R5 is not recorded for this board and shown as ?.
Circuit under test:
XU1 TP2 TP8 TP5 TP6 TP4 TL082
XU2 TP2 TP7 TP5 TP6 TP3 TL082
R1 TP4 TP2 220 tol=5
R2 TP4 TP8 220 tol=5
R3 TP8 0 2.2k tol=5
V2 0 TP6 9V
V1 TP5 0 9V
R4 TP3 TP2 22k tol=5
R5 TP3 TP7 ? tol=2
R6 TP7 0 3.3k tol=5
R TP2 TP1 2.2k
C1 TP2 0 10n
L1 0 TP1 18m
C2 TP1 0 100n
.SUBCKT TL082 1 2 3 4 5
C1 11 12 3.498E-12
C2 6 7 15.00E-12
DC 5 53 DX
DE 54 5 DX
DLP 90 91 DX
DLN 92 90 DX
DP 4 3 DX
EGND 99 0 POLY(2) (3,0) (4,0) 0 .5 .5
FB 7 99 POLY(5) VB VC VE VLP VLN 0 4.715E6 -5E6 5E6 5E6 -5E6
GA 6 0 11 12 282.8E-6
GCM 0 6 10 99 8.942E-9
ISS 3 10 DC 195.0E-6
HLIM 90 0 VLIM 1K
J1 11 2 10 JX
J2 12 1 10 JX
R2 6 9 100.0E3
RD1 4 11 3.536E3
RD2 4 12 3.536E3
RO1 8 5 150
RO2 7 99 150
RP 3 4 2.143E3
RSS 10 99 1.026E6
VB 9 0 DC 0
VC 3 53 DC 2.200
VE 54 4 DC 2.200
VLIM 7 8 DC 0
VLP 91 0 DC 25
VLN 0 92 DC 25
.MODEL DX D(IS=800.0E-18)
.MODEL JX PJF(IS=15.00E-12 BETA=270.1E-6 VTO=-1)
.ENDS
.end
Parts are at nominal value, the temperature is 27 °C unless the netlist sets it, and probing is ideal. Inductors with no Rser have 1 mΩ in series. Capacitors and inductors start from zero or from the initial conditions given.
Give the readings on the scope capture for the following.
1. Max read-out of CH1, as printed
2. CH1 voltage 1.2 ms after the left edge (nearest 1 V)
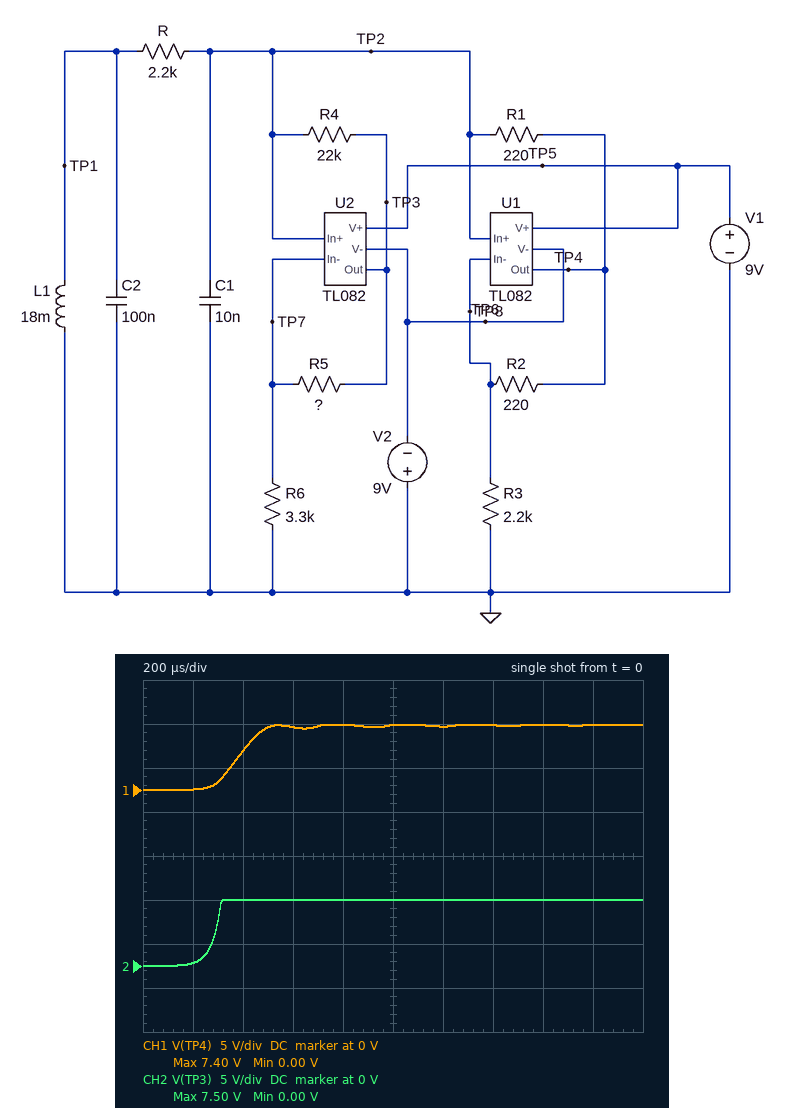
7.40 V
7 V
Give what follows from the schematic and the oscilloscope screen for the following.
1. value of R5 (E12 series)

18 kΩ
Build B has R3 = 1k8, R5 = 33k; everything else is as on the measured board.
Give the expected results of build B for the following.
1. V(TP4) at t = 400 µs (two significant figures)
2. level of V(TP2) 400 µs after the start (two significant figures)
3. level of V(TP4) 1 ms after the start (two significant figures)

7.4 V
6.7 V
7.4 V
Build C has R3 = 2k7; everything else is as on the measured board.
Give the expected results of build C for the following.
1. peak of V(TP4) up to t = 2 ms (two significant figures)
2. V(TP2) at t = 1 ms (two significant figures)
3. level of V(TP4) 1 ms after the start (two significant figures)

3.2 V
2.3 V
2.5 V
